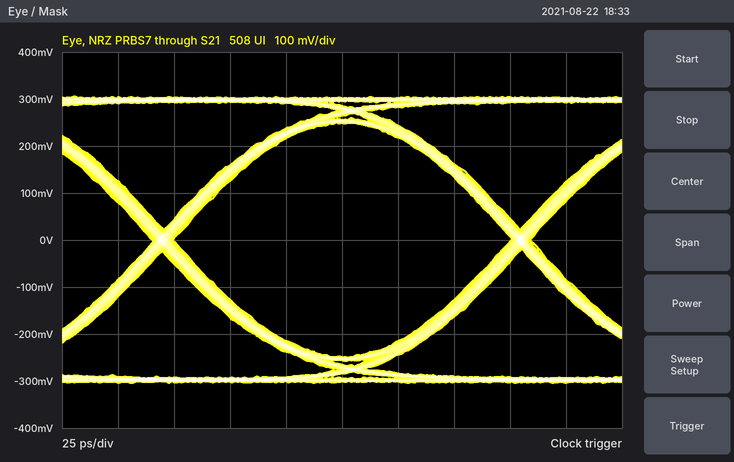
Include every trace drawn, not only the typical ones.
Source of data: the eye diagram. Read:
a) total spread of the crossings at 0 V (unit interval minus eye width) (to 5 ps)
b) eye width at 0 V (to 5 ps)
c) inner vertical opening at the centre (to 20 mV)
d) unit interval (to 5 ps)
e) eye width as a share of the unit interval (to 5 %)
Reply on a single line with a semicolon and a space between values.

10 ps; 150 ps; 500 mV; 160 ps; 95 %
